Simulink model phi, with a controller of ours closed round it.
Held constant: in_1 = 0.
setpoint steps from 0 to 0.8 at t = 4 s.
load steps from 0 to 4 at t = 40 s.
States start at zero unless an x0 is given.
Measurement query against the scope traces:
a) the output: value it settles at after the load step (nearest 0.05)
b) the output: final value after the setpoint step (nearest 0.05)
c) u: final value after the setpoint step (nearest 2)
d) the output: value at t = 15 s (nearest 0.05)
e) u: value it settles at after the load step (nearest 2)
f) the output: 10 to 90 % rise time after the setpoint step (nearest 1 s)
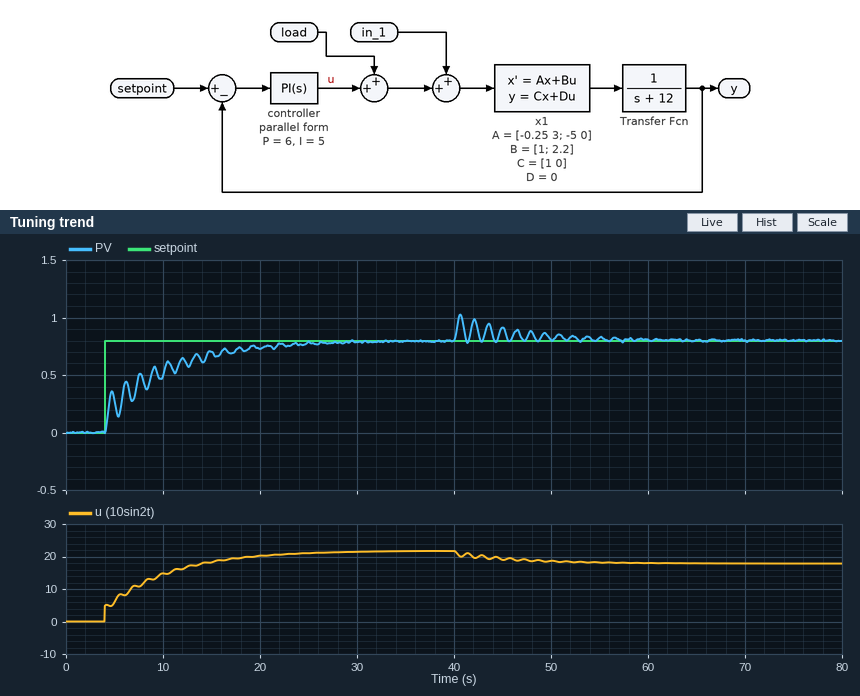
0.80
0.80
22
0.70
18
12 s
